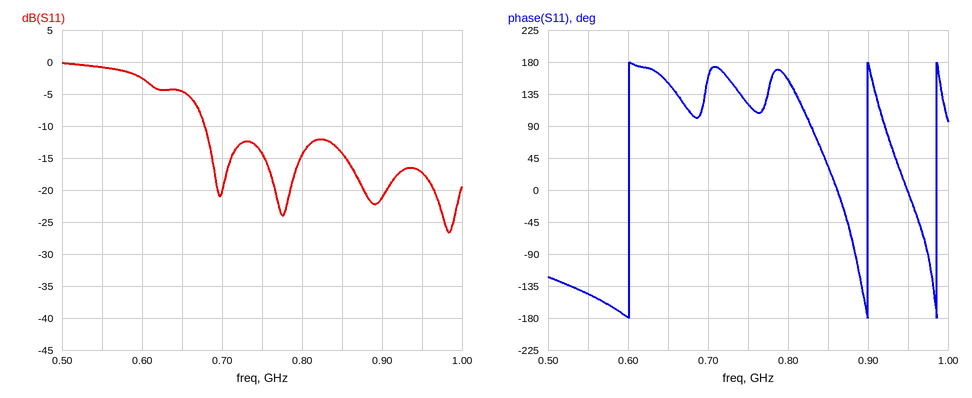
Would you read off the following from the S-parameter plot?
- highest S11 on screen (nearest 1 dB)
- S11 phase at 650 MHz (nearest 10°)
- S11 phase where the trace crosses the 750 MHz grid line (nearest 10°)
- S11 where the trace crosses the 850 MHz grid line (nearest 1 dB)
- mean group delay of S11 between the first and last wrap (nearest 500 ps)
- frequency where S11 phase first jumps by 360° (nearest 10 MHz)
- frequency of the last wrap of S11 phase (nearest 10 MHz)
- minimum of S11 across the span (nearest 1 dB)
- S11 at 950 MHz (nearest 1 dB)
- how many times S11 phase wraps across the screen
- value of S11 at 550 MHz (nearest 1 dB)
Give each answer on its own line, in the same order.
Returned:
0 dB
150°
120°
-14 dB
5.0 ns
600 MHz
990 MHz
-27 dB
-17 dB
3
-1 dB
